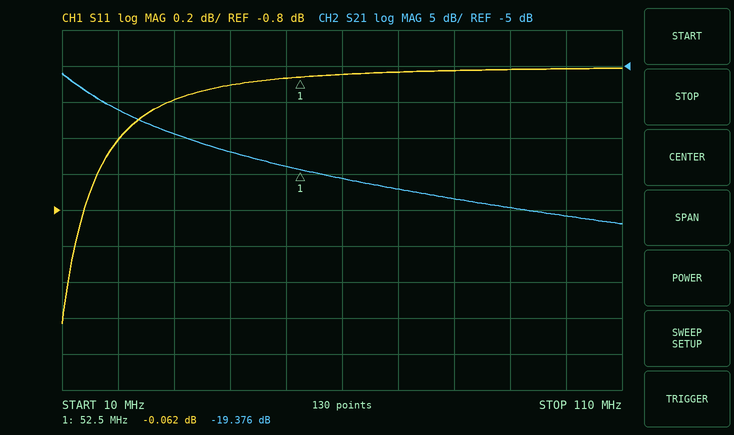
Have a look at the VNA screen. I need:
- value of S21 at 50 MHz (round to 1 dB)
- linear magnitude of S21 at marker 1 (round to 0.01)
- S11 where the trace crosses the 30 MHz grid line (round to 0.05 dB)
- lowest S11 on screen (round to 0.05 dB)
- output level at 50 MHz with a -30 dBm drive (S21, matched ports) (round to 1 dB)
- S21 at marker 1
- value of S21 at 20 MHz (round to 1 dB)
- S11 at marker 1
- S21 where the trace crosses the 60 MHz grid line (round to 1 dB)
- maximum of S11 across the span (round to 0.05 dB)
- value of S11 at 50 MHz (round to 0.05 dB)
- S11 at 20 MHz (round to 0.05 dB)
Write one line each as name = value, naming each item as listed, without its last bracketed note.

value of S21 at 50 MHz = -19 dB
linear magnitude of S21 at marker 1 = 0.11
S11 where the trace crosses the 30 MHz grid line = -0.20 dB
lowest S11 on screen = -1.45 dB
output level at 50 MHz with a -30 dBm drive (S21, matched ports) = -49 dBm
S21 at marker 1 = -19.376 dB
value of S21 at 20 MHz = -11 dB
S11 at marker 1 = -0.062 dB
S21 where the trace crosses the 60 MHz grid line = -21 dB
maximum of S11 across the span = 0.00 dB
value of S11 at 50 MHz = -0.05 dB
S11 at 20 MHz = -0.40 dB
